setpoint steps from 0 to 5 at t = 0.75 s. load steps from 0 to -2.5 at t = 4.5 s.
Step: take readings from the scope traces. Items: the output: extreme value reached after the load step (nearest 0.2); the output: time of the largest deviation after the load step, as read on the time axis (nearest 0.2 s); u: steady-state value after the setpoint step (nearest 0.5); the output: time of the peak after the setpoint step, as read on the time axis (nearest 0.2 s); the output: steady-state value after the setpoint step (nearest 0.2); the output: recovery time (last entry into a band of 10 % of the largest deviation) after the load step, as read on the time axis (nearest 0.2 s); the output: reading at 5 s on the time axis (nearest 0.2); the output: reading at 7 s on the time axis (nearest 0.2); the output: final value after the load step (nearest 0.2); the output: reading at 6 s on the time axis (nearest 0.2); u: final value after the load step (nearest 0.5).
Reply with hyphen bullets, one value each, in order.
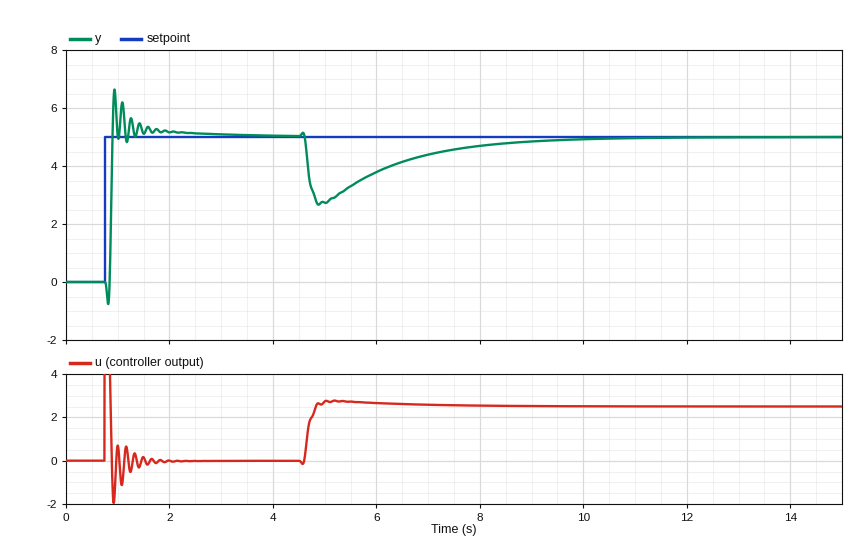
- 2.6
- 4.8 s
- 0.0
- 1.0 s
- 5.0
- 8.4 s
- 2.8
- 4.4
- 5.0
- 3.8
- 2.5
